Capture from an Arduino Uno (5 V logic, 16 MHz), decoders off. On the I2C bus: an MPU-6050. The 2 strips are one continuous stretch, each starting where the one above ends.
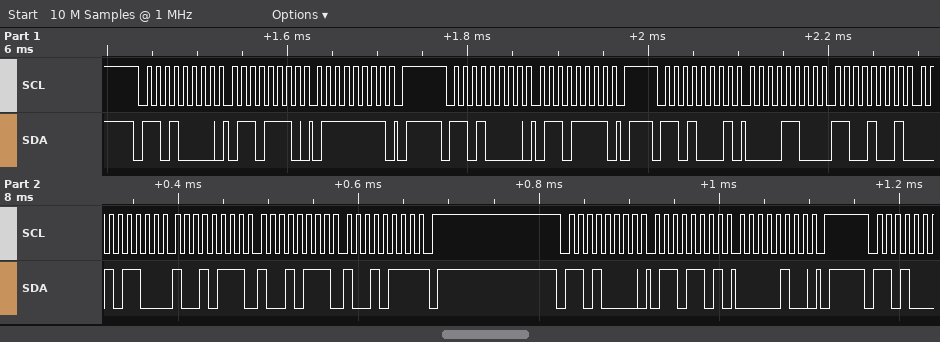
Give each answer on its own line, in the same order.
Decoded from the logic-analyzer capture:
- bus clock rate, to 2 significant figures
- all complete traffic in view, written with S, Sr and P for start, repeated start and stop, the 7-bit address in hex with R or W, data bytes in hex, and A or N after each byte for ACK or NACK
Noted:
100 kHz
S 68W A 6E A 7F A P S 68W A 6F A P S 68R A 0C A C9 A 2C A 97 A 97 A 97 N P S 68W A 6D A 04 A P
